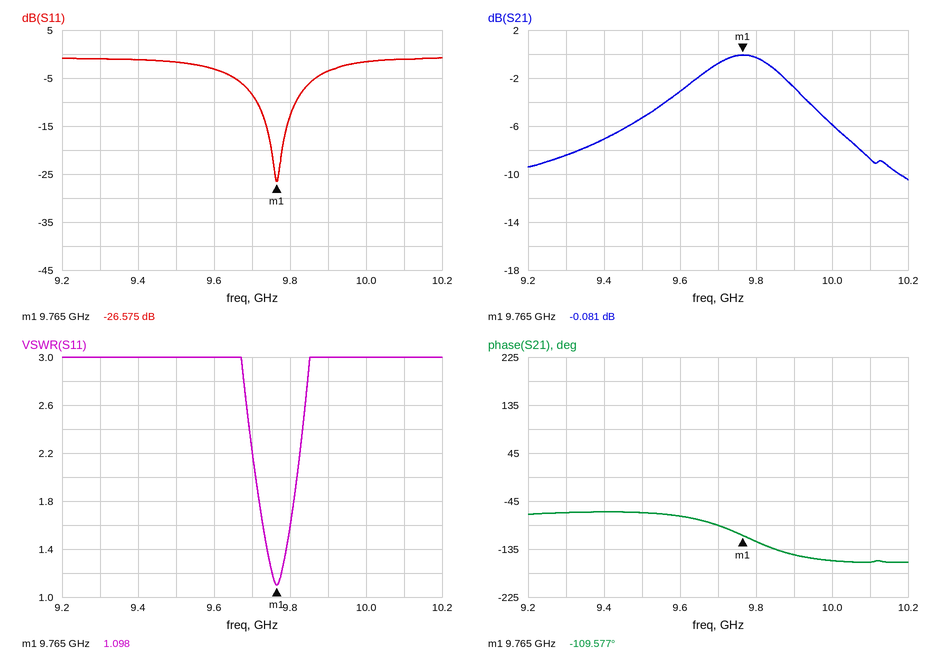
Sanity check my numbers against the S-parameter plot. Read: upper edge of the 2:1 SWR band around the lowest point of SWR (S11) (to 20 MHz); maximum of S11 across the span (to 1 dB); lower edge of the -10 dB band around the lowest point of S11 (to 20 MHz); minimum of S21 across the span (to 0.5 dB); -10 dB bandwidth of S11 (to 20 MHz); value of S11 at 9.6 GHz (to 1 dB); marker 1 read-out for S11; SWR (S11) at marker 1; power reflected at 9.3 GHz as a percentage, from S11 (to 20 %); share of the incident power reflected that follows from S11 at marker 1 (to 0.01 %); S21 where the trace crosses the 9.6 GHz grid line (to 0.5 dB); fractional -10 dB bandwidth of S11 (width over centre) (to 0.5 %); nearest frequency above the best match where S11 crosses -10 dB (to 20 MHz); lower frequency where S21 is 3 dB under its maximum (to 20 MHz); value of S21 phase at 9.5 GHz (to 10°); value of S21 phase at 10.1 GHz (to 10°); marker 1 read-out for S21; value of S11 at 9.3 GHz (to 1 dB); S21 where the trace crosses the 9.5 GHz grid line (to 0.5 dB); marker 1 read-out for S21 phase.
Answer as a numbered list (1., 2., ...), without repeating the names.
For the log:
1. 9.82 GHz
2. -1 dB
3. 9.72 GHz
4. -10.5 dB
5. 100 MHz
6. -3 dB
7. -26.575 dB
8. 1.098
9. 80 %
10. 0.22 %
11. -3.0 dB
12. 1.0 %
13. 9.82 GHz
14. 9.60 GHz
15. -70°
16. -160°
17. -0.081 dB
18. -1 dB
19. -5.5 dB
20. -109.577°
